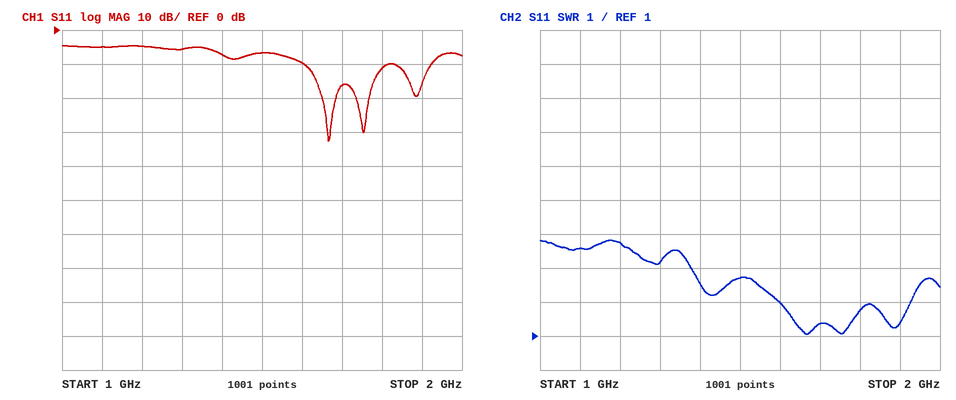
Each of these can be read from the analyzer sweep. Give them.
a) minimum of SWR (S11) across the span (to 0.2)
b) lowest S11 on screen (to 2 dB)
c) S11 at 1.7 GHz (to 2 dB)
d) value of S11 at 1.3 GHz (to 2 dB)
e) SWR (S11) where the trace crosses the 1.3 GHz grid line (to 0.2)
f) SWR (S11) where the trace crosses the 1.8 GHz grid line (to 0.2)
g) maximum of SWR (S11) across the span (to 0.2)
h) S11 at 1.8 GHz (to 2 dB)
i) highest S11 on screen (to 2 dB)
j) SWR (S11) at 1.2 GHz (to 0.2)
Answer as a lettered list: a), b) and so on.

a) 1.0
b) -32 dB
c) -16 dB
d) -6 dB
e) 3.2
f) 1.8
g) 3.8
h) -12 dB
i) -4 dB
j) 3.8
